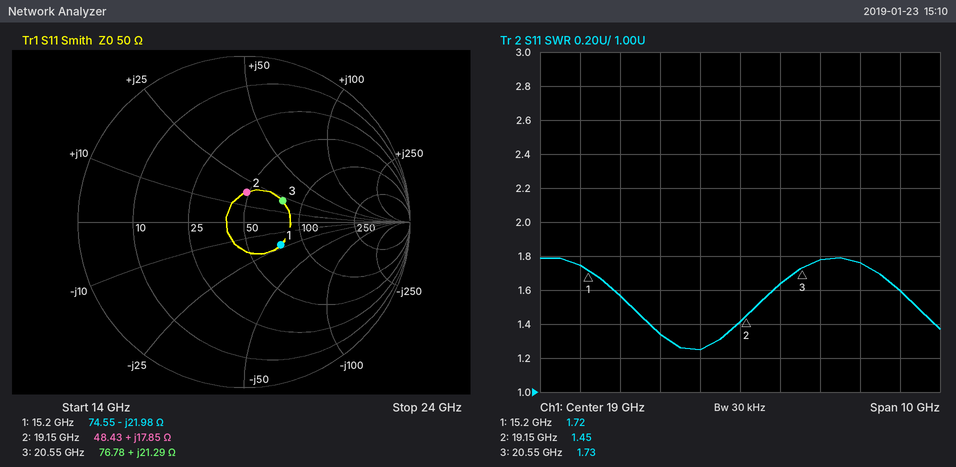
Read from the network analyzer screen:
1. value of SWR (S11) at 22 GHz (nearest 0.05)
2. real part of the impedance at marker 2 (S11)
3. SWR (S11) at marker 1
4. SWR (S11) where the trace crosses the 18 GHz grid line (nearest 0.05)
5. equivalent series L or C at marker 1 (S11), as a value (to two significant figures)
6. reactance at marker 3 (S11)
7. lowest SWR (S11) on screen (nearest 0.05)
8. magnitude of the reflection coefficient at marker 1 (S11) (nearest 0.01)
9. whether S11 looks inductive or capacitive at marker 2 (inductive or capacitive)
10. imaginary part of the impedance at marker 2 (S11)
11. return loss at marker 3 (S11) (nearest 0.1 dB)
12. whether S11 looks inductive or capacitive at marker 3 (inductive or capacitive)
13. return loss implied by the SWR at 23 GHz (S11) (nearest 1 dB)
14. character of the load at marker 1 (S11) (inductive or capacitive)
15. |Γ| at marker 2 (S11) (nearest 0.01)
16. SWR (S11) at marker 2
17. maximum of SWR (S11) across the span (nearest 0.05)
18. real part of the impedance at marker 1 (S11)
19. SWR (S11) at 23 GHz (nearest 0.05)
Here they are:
1.75
48.43 Ω
1.72
1.25
480 fF
+21.29 Ω
1.25
0.26
inductive
+17.85 Ω
11.5 dB
inductive
13 dB
capacitive
0.18
1.45
1.80
74.55 Ω
1.60
